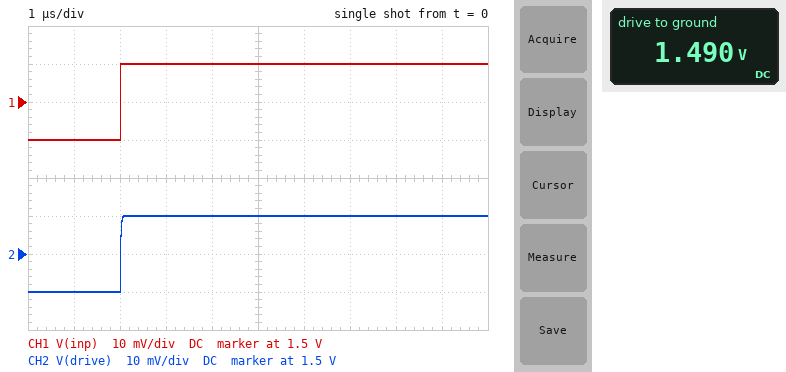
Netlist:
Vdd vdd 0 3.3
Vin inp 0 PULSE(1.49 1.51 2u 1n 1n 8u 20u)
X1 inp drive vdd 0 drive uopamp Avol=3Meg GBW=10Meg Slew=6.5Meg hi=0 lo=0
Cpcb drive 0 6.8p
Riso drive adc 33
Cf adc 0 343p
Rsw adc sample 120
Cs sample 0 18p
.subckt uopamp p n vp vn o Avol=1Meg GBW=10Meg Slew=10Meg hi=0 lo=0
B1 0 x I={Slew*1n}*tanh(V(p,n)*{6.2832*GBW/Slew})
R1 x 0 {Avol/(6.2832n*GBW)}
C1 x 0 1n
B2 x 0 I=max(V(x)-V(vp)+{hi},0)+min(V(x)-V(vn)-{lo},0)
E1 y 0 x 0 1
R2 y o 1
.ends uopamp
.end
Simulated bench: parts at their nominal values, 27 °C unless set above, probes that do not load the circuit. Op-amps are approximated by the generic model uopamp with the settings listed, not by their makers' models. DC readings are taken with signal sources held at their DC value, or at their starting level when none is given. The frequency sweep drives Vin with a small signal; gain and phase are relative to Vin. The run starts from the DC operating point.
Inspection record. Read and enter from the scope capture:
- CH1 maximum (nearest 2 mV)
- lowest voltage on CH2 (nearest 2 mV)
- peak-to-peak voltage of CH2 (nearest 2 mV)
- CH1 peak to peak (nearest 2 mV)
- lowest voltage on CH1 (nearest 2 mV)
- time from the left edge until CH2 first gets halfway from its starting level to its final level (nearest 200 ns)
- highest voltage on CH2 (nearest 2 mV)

1.510 V
1.490 V
20 mV
20 mV
1.490 V
2.0 µs
1.510 V
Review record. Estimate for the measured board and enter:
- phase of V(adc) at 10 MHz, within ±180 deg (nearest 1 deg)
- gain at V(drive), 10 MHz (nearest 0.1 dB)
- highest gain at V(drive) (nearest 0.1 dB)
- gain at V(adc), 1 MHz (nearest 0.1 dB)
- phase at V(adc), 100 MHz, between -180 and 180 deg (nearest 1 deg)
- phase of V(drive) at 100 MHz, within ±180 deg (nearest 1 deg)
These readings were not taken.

-82 deg
-3.0 dB
0 dB
-0.1 dB
-166 deg
-85 deg
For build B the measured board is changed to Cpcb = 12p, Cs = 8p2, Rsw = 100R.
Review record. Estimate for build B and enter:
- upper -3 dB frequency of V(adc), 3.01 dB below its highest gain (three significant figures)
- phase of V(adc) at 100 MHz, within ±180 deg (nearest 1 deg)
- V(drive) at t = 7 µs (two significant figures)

7.45 MHz
-167 deg
1.5 V
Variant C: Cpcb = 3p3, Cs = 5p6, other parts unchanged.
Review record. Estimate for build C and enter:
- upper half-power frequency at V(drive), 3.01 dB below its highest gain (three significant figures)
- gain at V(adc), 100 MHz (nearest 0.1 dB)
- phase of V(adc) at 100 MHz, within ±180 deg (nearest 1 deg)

10.0 MHz
-37.5 dB
-167 deg
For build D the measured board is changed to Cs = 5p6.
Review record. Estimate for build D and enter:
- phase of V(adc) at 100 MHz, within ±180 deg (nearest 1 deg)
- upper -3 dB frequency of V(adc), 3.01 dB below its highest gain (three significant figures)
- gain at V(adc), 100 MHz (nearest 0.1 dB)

-167 deg
7.48 MHz
-37.5 dB
